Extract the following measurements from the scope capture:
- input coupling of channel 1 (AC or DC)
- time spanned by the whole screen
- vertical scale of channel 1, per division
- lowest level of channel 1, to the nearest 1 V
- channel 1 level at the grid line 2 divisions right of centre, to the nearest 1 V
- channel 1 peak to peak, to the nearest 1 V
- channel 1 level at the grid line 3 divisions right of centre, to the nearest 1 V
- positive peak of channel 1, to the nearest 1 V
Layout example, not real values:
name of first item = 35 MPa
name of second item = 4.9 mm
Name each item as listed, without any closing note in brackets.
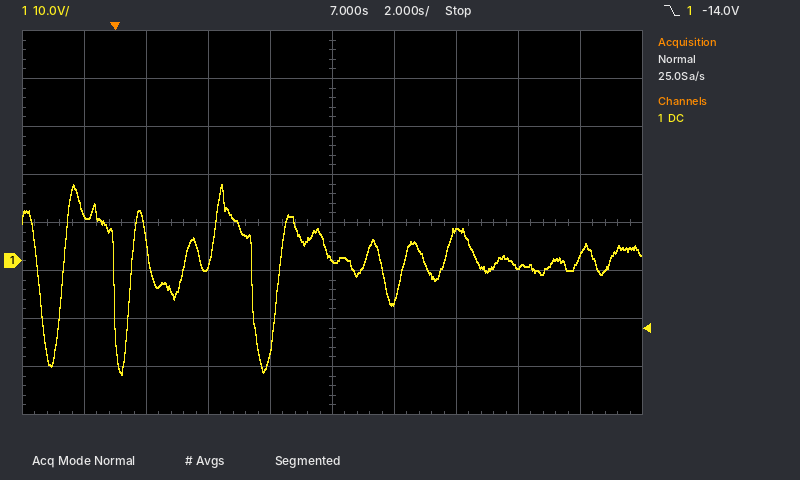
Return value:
input coupling of channel 1 = DC
time spanned by the whole screen = 20 s
vertical scale of channel 1, per division = 10 V
lowest level of channel 1, to the nearest 1 V = -24 V
channel 1 level at the grid line 2 divisions right of centre, to the nearest 1 V = 6 V
channel 1 peak to peak, to the nearest 1 V = 40 V
channel 1 level at the grid line 3 divisions right of centre, to the nearest 1 V = -1 V
positive peak of channel 1, to the nearest 1 V = 16 V
